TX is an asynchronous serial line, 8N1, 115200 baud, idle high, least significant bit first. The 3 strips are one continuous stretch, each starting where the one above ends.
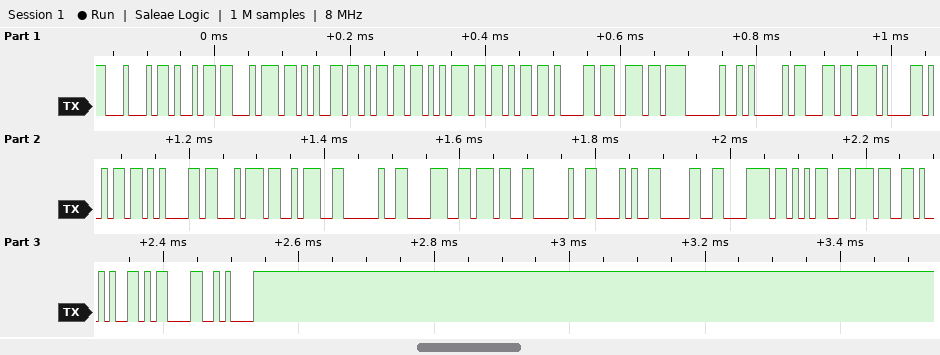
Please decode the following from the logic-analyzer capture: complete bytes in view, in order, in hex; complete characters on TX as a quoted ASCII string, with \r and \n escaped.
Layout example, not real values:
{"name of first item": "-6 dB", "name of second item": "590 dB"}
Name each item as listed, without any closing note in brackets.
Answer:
{"complete bytes in view, in order, in hex": "44 69 74 65 6D 75 6B 61 6E 20 41 6C 61 6D 61 74 3A 20 38 37 20 28 30 78 35 37 29 0D 0A", "complete characters on TX as a quoted ASCII string, with \\r and \\n escaped": "\"Ditemukan Alamat: 87 (0x57)\\r\\n\""}
